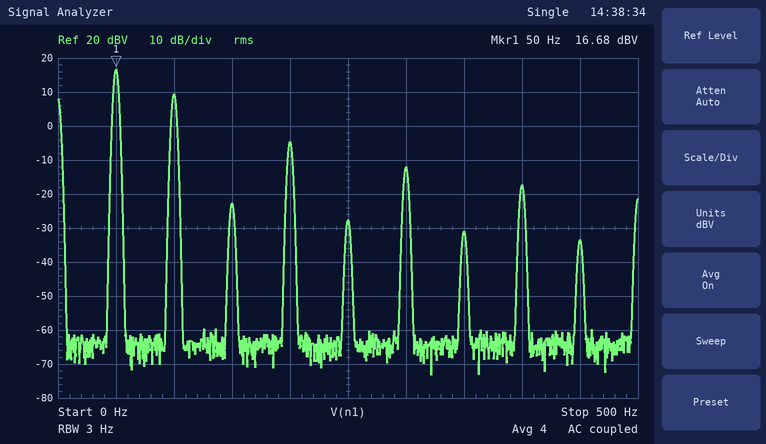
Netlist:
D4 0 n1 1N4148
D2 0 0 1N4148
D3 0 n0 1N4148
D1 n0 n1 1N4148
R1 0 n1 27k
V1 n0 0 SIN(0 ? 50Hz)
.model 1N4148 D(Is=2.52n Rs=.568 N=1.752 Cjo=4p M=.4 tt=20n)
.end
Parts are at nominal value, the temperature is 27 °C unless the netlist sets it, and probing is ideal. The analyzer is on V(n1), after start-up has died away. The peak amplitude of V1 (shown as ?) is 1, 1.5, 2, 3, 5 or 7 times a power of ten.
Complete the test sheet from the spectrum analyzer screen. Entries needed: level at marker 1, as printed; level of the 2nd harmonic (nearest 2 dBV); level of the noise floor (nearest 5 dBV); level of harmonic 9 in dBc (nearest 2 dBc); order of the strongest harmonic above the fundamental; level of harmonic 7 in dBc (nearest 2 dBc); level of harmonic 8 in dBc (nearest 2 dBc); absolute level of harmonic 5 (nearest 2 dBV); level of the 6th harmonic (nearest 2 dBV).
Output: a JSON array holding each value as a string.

["16.68 dBV", "10 dBV", "-65 dBV", "-50 dBc", "2", "-48 dBc", "-34 dBc", "-28 dBV", "-12 dBV"]
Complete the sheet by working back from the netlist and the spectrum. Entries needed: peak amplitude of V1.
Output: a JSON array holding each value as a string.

["20 V"]
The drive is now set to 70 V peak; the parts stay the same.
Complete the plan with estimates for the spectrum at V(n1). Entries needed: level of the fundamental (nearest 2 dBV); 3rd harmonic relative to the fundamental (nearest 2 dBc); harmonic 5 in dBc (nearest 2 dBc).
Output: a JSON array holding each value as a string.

["28 dBV", "-50 dBc", "-54 dBc"]
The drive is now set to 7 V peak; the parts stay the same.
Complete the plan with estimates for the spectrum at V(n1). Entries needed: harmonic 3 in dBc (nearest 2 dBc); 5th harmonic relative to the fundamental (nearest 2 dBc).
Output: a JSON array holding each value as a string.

["-30 dBc", "-36 dBc"]
